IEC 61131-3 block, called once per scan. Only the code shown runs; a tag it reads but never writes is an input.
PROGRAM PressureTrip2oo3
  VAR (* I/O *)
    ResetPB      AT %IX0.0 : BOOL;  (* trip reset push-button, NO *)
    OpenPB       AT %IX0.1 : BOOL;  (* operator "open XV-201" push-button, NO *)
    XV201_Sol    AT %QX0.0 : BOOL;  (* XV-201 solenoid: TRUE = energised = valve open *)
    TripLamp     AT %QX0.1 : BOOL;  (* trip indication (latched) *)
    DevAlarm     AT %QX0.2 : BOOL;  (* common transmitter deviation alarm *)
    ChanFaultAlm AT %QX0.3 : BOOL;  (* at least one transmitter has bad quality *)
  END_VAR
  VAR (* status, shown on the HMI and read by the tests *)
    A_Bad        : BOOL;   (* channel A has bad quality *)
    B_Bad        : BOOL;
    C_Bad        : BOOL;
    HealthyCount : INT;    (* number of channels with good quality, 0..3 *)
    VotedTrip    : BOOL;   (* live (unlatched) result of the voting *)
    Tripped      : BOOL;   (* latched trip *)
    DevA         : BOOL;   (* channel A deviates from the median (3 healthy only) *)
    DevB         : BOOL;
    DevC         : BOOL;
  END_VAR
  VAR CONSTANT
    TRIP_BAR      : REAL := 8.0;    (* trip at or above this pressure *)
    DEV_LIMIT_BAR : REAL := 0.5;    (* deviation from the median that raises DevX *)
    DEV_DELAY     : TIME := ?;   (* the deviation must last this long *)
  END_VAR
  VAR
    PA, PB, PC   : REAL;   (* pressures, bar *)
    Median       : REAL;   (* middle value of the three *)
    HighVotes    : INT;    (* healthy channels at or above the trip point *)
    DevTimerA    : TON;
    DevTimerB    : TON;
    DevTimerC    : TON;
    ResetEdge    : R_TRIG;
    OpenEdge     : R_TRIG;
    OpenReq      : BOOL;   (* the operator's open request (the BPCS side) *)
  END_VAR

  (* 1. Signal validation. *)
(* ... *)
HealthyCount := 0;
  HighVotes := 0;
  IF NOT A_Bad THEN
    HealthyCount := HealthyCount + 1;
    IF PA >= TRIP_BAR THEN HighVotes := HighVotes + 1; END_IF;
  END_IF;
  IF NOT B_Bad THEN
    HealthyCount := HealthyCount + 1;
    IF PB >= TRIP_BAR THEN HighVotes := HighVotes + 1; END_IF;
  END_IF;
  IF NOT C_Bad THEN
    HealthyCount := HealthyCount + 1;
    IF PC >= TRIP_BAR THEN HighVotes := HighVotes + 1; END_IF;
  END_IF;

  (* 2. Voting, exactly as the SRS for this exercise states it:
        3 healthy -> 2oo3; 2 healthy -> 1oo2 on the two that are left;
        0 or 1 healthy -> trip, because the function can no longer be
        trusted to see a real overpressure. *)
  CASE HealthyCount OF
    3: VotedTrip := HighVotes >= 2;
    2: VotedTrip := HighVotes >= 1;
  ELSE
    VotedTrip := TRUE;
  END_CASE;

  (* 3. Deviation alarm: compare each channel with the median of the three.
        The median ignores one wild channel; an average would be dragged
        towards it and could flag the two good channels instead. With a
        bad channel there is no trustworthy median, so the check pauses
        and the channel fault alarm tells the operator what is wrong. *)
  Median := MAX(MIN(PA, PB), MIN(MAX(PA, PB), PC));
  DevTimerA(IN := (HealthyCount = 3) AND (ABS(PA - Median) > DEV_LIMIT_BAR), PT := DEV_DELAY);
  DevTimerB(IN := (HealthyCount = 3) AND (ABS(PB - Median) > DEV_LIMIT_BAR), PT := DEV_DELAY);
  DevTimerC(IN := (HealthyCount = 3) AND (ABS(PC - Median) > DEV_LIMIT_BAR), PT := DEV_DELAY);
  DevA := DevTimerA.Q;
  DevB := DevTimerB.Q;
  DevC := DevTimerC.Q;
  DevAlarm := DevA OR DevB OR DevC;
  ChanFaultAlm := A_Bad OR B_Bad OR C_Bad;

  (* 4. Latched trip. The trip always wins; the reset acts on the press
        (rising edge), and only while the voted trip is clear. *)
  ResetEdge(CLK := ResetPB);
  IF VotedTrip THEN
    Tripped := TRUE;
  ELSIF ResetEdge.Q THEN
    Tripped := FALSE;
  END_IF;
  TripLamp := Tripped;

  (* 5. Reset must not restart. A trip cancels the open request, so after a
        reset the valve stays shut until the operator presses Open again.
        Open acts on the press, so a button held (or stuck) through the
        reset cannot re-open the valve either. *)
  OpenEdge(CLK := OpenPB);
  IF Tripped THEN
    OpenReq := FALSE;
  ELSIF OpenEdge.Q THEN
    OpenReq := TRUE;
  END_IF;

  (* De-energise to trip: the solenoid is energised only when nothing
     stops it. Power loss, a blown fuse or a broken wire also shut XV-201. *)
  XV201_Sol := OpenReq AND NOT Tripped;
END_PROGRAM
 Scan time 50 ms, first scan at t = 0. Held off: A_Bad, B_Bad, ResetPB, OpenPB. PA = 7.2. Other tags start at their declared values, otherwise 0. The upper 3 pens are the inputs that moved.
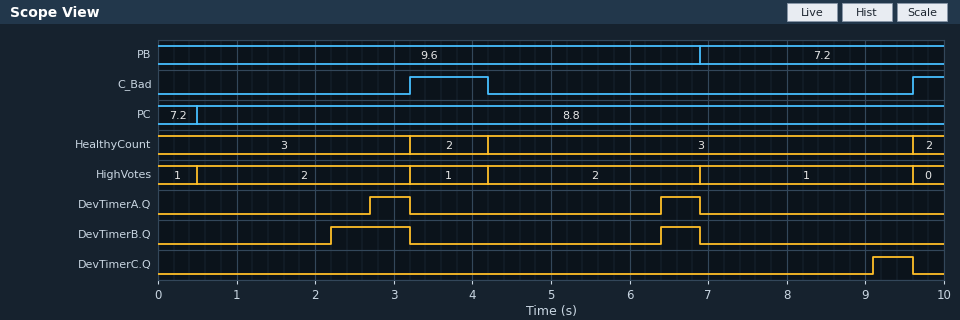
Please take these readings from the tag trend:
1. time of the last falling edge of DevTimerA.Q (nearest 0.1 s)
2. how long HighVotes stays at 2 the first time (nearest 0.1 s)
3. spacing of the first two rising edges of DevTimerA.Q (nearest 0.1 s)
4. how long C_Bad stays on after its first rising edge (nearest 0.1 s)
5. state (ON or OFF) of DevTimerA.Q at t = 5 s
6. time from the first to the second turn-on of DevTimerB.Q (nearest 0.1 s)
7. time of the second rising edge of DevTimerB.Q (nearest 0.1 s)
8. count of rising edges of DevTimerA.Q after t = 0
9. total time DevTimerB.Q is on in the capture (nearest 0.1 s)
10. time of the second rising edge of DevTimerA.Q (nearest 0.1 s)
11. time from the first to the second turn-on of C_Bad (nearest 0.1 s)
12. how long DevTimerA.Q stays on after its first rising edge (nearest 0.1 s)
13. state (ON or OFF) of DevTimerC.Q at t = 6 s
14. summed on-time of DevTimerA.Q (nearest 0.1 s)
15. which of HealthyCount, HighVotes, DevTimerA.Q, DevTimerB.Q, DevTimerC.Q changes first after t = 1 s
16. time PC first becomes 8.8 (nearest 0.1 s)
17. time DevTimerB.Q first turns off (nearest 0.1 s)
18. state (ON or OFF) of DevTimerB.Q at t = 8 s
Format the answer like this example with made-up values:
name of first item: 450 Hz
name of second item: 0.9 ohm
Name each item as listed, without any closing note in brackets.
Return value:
time of the last falling edge of DevTimerA.Q: 6.9 s
how long HighVotes stays at 2 the first time: 2.7 s
spacing of the first two rising edges of DevTimerA.Q: 3.7 s
how long C_Bad stays on after its first rising edge: 1.0 s
state (ON or OFF) of DevTimerA.Q at t = 5 s: OFF
time from the first to the second turn-on of DevTimerB.Q: 4.2 s
time of the second rising edge of DevTimerB.Q: 6.4 s
count of rising edges of DevTimerA.Q after t = 0: 2
total time DevTimerB.Q is on in the capture: 1.5 s
time of the second rising edge of DevTimerA.Q: 6.4 s
time from the first to the second turn-on of C_Bad: 6.4 s
how long DevTimerA.Q stays on after its first rising edge: 0.5 s
state (ON or OFF) of DevTimerC.Q at t = 6 s: OFF
summed on-time of DevTimerA.Q: 1.0 s
which of HealthyCount, HighVotes, DevTimerA.Q, DevTimerB.Q, DevTimerC.Q changes first after t = 1 s: DevTimerB.Q
time PC first becomes 8.8: 0.5 s
time DevTimerB.Q first turns off: 3.2 s
state (ON or OFF) of DevTimerB.Q at t = 8 s: OFF
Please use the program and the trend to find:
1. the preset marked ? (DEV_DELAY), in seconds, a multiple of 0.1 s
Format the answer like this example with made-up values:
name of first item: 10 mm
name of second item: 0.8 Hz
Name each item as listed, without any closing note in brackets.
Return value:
the preset marked ? (DEV_DELAY), in seconds, a multiple of 0.1 s: 2.2 s
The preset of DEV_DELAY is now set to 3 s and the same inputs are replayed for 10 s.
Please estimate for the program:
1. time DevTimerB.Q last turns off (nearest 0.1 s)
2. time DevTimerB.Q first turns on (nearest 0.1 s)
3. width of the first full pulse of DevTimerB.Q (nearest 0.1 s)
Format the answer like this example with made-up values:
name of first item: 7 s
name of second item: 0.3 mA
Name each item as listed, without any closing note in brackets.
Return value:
time DevTimerB.Q last turns off: 3.2 s
time DevTimerB.Q first turns on: 3.0 s
width of the first full pulse of DevTimerB.Q: 0.2 s
